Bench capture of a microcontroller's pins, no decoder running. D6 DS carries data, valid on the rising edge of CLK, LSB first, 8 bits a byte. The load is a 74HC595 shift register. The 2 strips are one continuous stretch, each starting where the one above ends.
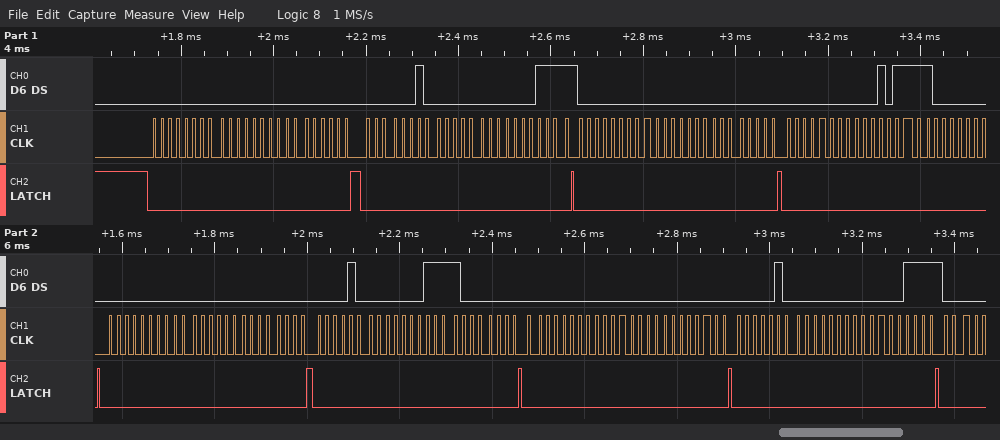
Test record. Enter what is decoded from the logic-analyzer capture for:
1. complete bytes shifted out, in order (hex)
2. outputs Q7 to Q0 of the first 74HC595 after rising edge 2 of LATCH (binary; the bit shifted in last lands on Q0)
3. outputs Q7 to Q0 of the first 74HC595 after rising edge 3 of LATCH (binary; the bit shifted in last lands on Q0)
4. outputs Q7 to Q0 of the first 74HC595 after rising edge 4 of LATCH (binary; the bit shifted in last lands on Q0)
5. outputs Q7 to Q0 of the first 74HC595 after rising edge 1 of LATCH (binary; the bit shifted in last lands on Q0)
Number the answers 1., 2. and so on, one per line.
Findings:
1. 00 00 00 40 00 F0 00 00 00 00 E8 01 00 00 00 10 E0 01 00 00 00 20 00 F0
2. 00001111
3. 00000000
4. 10000000
5. 00000000
